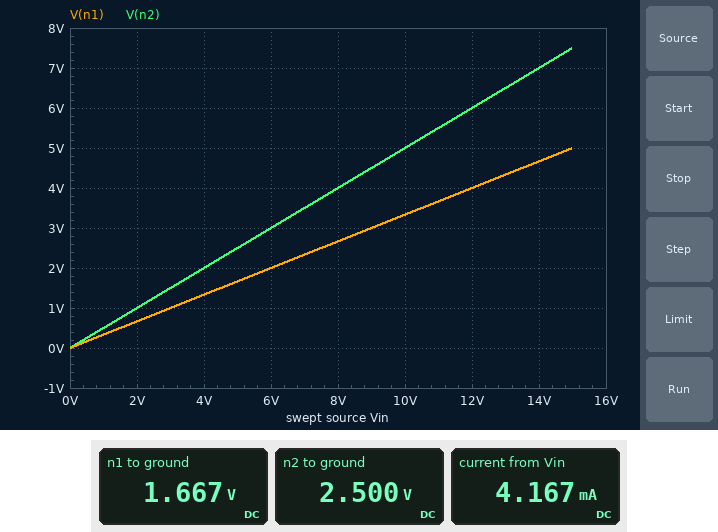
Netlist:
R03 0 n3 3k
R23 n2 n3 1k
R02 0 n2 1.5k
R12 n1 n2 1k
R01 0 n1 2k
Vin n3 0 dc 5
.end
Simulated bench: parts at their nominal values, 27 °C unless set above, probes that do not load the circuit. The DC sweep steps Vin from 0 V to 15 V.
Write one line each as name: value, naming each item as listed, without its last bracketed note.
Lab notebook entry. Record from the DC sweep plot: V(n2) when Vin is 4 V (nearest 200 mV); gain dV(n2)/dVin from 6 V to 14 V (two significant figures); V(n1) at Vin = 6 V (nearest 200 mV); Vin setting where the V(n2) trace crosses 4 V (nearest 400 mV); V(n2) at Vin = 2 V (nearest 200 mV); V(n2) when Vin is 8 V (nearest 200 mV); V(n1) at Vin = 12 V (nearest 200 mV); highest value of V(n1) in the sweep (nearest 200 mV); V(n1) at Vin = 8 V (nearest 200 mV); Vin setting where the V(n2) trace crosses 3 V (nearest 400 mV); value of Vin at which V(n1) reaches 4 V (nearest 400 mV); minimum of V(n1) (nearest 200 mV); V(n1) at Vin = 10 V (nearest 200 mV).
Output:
V(n2) when Vin is 4 V: 2.0 V
gain dV(n2)/dVin from 6 V to 14 V: 0.50 V/V
V(n1) at Vin = 6 V: 2.0 V
Vin setting where the V(n2) trace crosses 4 V: 8.0 V
V(n2) at Vin = 2 V: 1.0 V
V(n2) when Vin is 8 V: 4.0 V
V(n1) at Vin = 12 V: 4.0 V
highest value of V(n1) in the sweep: 5.0 V
V(n1) at Vin = 8 V: 2.6 V
Vin setting where the V(n2) trace crosses 3 V: 6.0 V
value of Vin at which V(n1) reaches 4 V: 12.0 V
minimum of V(n1): 0 V
V(n1) at Vin = 10 V: 3.4 V
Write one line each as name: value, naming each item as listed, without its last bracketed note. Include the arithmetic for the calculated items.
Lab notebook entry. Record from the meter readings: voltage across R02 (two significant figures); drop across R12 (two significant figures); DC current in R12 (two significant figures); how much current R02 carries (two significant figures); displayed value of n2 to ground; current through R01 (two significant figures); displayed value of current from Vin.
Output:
voltage across R02: 2.5 V = 2.5 V
drop across R12: 2.5 V - 1.667 V = 830 mV
DC current in R12: (2.5 V - 1.667 V) / 1 kΩ = 830 µA
how much current R02 carries: (2.5 V) / 1.5 kΩ = 1.7 mA
displayed value of n2 to ground: 2.500 V
current through R01: (1.667 V) / 2 kΩ = 830 µA
displayed value of current from Vin: 4.167 mA
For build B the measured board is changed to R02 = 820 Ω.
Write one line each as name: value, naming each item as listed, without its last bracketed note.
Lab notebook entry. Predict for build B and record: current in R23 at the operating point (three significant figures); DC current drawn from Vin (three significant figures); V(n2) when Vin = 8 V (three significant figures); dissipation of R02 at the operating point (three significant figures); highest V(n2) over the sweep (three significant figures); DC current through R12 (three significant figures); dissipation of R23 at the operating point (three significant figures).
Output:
current in R23 at the operating point: 3.04 mA
DC current drawn from Vin: 4.71 mA
V(n2) when Vin = 8 V: 3.13 V
dissipation of R02 at the operating point: 4.68 mW
highest V(n2) over the sweep: 5.88 V
DC current through R12: 653 µA
dissipation of R23 at the operating point: 9.25 mW
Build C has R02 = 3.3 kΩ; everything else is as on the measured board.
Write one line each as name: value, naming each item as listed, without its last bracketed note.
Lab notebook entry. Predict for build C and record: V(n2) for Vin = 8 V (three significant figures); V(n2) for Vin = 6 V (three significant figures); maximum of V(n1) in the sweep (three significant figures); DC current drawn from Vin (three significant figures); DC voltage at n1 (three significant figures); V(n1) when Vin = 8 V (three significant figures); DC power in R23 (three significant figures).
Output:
V(n2) for Vin = 8 V: 4.89 V
V(n2) for Vin = 6 V: 3.67 V
maximum of V(n1) in the sweep: 6.11 V
DC current drawn from Vin: 3.61 mA
DC voltage at n1: 2.04 V
V(n1) when Vin = 8 V: 3.26 V
DC power in R23: 3.78 mW
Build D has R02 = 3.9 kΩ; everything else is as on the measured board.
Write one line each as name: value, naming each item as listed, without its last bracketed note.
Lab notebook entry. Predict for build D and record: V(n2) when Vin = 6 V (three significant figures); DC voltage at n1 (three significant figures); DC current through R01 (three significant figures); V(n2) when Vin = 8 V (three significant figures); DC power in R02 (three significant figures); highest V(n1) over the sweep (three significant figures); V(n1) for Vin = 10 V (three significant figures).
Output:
V(n2) when Vin = 6 V: 3.77 V
DC voltage at n1: 2.10 V
DC current through R01: 1.05 mA
V(n2) when Vin = 8 V: 5.03 V
DC power in R02: 2.54 mW
highest V(n1) over the sweep: 6.29 V
V(n1) for Vin = 10 V: 4.19 V
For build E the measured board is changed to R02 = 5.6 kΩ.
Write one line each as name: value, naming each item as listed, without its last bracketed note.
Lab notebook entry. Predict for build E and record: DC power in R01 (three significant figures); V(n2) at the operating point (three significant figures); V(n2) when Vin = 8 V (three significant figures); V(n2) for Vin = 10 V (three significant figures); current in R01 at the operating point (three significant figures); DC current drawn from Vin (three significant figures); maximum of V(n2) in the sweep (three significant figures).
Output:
DC power in R01: 2.43 mW
V(n2) at the operating point: 3.31 V
V(n2) when Vin = 8 V: 5.29 V
V(n2) for Vin = 10 V: 6.61 V
current in R01 at the operating point: 1.10 mA
DC current drawn from Vin: 3.36 mA
maximum of V(n2) in the sweep: 9.92 V
